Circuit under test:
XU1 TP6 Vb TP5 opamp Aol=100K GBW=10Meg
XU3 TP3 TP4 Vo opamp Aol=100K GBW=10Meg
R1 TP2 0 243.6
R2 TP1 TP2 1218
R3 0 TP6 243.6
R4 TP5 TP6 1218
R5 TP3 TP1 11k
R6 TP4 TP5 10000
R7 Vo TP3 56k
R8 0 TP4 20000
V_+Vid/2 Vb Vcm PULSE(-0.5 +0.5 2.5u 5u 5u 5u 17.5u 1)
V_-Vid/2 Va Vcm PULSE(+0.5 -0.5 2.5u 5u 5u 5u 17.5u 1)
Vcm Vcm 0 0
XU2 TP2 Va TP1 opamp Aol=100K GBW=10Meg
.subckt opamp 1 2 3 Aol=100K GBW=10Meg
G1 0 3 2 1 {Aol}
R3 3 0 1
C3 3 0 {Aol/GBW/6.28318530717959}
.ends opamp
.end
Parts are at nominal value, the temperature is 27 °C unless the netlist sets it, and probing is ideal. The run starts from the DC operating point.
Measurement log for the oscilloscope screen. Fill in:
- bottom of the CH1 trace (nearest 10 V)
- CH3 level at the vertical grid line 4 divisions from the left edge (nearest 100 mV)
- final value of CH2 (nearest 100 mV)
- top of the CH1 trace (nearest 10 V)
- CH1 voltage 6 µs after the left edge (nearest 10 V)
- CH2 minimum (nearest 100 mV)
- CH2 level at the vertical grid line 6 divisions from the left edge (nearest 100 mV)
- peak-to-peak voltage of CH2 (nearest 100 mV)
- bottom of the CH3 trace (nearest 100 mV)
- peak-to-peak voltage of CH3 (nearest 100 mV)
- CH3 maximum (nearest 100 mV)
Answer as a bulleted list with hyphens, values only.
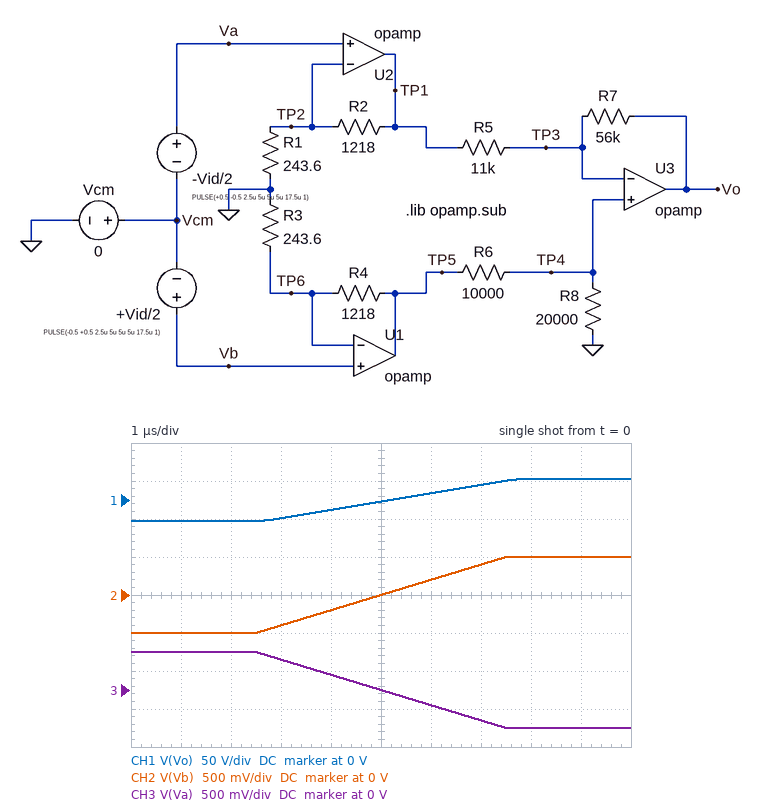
- -30 V
- 200 mV
- 500 mV
- 30 V
- 10 V
- -500 mV
- 200 mV
- 1.0 V
- -500 mV
- 1.0 V
- 500 mV
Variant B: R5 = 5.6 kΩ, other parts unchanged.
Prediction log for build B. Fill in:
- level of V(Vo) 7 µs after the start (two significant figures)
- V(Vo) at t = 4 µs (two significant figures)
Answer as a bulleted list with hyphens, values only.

- 36 V
- -26 V
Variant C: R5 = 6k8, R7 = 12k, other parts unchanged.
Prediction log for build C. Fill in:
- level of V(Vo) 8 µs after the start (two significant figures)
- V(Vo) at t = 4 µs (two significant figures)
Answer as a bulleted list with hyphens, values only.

- 11 V
- -4.9 V
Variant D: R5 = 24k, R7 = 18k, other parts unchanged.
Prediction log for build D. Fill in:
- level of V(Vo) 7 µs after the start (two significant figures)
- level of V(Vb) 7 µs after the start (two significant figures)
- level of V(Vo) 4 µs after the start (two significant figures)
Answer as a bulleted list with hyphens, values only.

- 4.3 V
- 400 mV
- -2.6 V
